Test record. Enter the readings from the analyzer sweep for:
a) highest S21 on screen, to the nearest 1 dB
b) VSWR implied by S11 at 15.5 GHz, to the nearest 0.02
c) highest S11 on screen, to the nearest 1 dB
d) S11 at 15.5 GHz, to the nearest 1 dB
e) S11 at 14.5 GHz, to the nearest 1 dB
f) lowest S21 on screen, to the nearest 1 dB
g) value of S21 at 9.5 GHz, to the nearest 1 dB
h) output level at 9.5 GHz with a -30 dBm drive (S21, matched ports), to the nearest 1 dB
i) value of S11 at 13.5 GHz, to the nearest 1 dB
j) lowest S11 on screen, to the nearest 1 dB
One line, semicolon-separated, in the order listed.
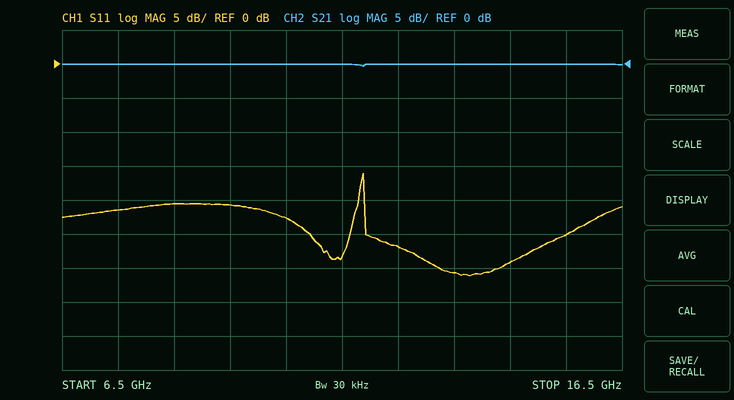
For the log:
0 dB; 1.12; -16 dB; -25 dB; -29 dB; 0 dB; 0 dB; -30 dBm; -31 dB; -31 dB
